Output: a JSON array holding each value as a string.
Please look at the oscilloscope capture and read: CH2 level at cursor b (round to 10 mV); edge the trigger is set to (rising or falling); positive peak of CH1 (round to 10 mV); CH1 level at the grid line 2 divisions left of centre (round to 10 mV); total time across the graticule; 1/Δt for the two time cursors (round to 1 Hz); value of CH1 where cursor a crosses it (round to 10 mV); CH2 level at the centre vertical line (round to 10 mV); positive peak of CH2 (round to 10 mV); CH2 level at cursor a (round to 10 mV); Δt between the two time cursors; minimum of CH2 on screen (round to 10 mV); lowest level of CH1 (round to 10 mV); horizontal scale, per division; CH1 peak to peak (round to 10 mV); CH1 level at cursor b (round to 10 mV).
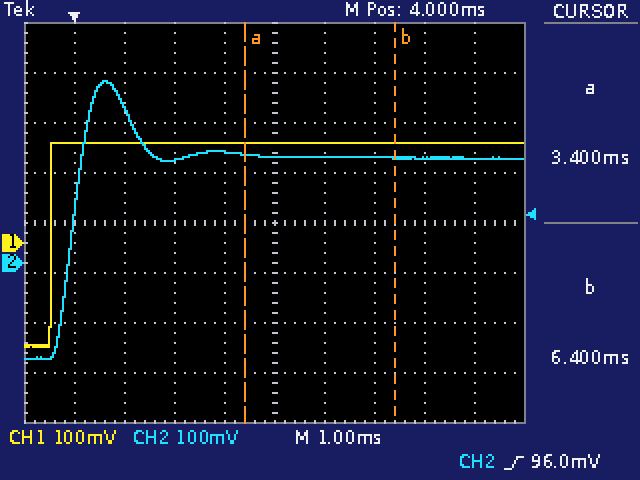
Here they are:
["210 mV", "rising", "200 mV", "200 mV", "10 ms", "333 Hz", "200 mV", "210 mV", "360 mV", "220 mV", "3.0 ms", "-190 mV", "-210 mV", "1 ms", "410 mV", "200 mV"]
